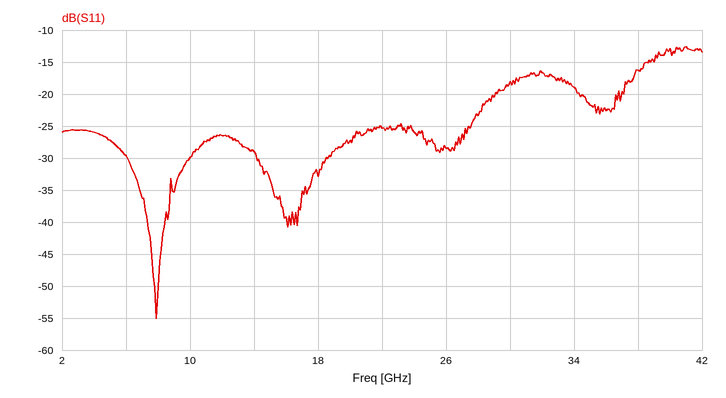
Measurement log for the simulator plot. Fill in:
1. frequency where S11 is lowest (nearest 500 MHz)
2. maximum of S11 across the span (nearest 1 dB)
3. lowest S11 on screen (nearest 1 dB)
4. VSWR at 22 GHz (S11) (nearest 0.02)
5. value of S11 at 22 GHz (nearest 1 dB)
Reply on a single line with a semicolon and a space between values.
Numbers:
8.0 GHz; -13 dB; -55 dB; 1.12; -25 dB
